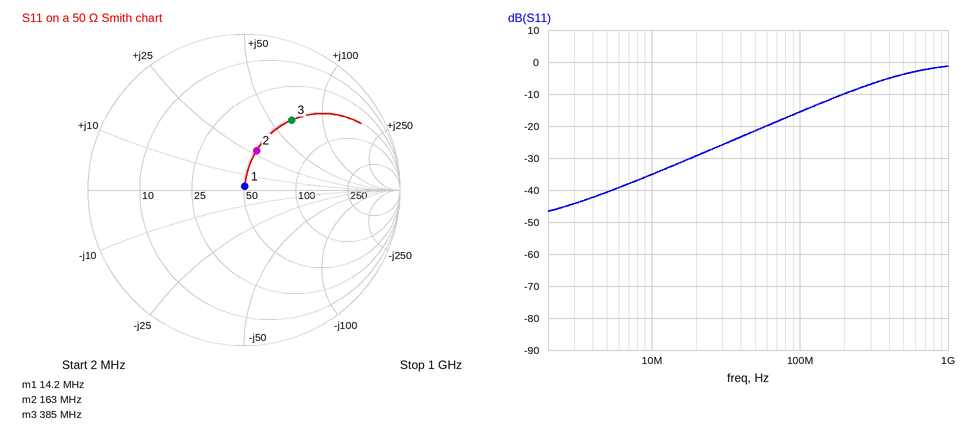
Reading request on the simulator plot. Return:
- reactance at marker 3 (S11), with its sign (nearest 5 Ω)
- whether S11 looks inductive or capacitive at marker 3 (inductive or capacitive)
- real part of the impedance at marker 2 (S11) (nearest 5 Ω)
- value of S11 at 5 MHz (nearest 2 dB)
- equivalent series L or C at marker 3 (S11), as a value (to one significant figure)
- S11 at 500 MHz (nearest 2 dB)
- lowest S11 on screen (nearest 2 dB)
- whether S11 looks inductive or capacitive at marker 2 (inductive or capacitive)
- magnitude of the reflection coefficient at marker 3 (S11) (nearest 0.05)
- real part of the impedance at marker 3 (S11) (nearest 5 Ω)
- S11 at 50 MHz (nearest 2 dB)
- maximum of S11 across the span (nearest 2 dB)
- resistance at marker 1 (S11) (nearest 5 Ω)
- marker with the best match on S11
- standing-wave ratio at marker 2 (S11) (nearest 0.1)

+65 Ω
inductive
50 Ω
-40 dB
30 nH
-4 dB
-46 dB
inductive
0.55
50 Ω
-22 dB
-2 dB
50 Ω
marker 1
1.7
